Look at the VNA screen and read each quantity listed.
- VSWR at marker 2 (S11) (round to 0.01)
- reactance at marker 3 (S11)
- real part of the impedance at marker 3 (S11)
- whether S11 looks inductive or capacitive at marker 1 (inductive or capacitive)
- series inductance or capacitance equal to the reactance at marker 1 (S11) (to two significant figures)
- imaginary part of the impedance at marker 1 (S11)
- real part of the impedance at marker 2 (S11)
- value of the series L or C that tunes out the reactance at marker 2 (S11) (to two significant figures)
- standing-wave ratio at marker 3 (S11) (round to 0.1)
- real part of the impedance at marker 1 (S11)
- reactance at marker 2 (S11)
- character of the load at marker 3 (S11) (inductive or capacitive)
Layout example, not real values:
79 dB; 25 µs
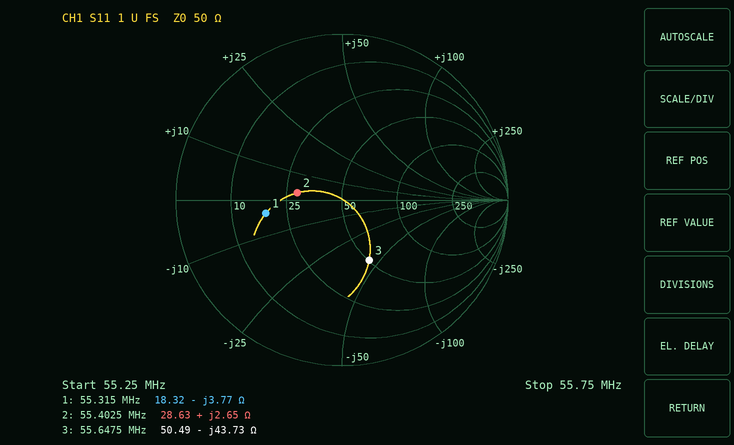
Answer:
1.75; -43.73 Ω; 50.49 Ω; capacitive; 760 pF; -3.77 Ω; 28.63 Ω; 1.1 nF; 2.3; 18.32 Ω; +2.65 Ω; capacitive
